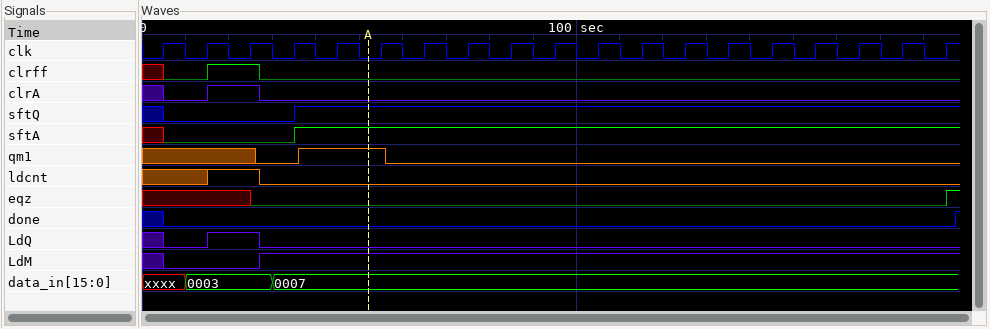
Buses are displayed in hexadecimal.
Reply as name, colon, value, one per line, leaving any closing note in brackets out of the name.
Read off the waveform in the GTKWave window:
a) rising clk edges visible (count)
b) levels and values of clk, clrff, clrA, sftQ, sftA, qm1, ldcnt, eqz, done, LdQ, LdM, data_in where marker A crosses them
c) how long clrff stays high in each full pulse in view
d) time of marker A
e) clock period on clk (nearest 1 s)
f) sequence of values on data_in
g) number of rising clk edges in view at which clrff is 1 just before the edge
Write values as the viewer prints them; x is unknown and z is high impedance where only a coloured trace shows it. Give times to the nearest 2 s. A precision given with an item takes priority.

rising clk edges visible: 19
levels and values of clk, clrff, clrA, sftQ, sftA, qm1, ldcnt, eqz, done, LdQ, LdM, data_in where marker A crosses them: clk=0, clrff=0, clrA=0, sftQ=1, sftA=1, qm1=1, ldcnt=0, eqz=0, done=0, LdQ=0, LdM=1, data_in=0007
how long clrff stays high in each full pulse in view: 12 s
time of marker A: 52 s
clock period on clk: 10 s
sequence of values on data_in: xxxx, 0003, 0007
number of rising clk edges in view at which clrff is 1 just before the edge: 1
